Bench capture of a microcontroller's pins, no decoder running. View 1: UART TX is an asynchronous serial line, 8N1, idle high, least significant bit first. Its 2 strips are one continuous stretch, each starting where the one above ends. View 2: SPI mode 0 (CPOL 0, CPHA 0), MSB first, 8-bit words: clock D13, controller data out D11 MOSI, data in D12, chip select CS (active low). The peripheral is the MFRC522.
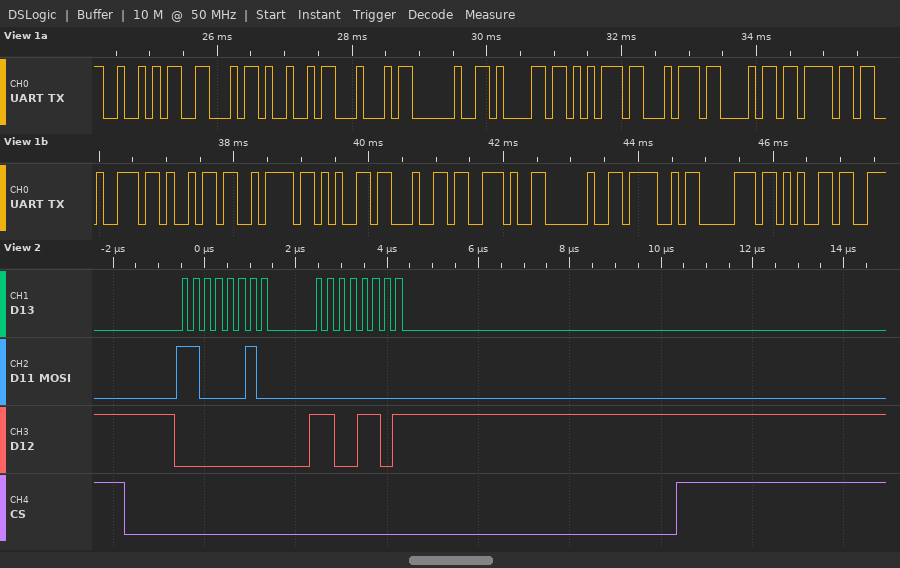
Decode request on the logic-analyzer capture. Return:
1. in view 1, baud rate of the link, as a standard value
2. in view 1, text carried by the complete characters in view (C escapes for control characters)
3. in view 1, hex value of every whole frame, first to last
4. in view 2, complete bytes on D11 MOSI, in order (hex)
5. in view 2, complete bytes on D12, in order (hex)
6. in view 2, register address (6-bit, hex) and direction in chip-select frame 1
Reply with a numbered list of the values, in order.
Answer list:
1. 9600 baud
2. "RFID authorized. Ope"
3. 52 46 49 44 20 61 75 74 68 6F 72 69 7A 65 64 2E 20 4F 70 65
4. C2 00
5. 00 CD
6. 0x21 read
